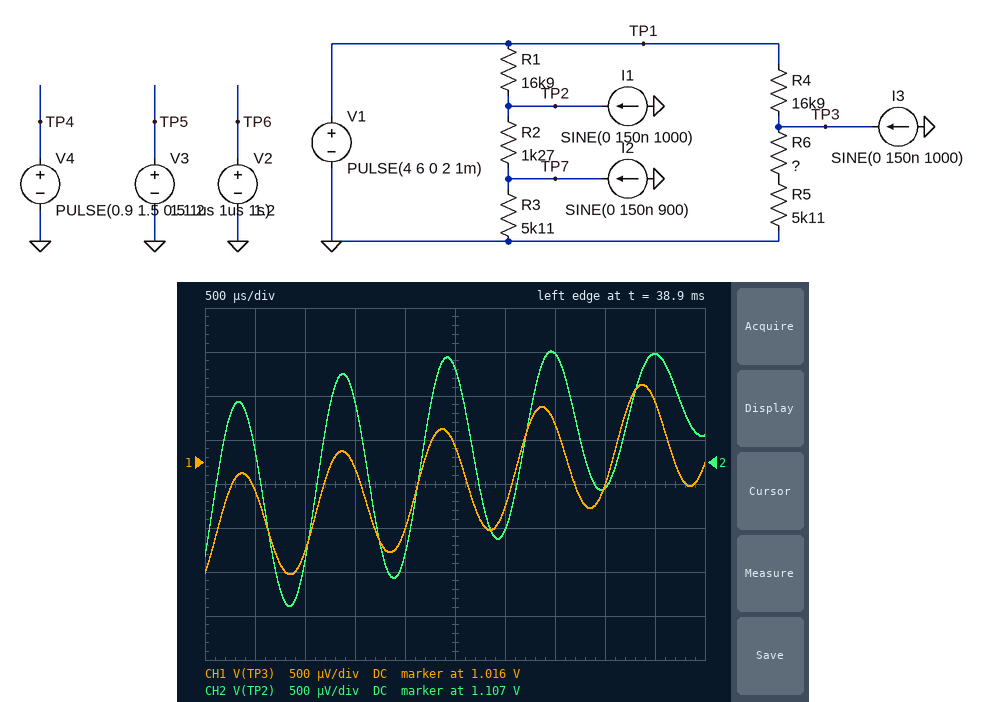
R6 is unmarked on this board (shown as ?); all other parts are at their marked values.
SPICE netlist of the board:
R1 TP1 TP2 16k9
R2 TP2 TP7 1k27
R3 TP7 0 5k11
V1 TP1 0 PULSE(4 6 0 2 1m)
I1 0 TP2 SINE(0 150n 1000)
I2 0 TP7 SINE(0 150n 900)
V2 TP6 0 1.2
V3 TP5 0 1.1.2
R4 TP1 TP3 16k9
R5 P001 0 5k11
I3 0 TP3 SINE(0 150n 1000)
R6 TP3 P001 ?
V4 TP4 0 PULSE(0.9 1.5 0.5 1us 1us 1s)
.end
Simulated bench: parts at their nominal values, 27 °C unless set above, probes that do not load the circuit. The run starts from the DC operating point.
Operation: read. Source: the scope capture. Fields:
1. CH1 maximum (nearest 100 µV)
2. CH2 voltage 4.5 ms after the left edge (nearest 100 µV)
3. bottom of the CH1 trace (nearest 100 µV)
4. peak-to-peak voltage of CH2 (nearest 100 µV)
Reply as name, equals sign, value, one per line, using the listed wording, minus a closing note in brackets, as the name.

CH1 maximum = 1.0164 V
CH2 voltage 4.5 ms after the left edge = 1.1087 V
bottom of the CH1 trace = 1.0142 V
peak-to-peak voltage of CH2 = 2.9 mV
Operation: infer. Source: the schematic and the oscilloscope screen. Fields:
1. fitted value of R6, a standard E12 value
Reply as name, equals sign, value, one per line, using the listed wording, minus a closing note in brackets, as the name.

fitted value of R6, a standard E12 value = 560 Ω
